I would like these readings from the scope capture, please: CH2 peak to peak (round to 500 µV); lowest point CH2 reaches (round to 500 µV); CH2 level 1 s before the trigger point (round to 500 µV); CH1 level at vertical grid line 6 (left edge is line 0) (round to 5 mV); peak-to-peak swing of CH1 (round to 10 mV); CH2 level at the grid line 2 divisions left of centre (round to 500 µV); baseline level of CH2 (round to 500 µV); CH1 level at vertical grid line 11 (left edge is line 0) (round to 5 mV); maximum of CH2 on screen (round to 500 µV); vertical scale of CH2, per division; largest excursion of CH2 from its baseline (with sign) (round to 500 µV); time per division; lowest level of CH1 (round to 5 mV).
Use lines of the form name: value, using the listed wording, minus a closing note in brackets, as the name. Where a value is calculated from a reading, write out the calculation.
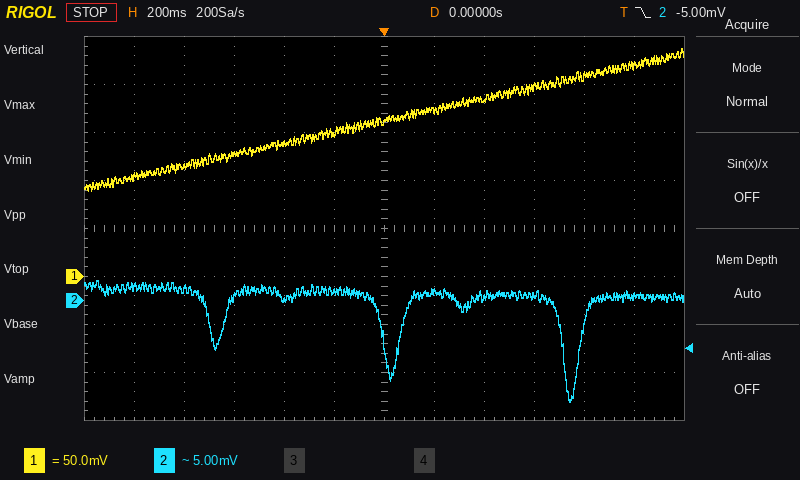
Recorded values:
CH2 peak to peak: 2.0 mV − (-10.5 mV) = 12.5 mV
lowest point CH2 reaches: -10.5 mV
CH2 level 1 s before the trigger point: 1.5 mV
CH1 level at vertical grid line 6 (left edge is line 0): 160 mV
peak-to-peak swing of CH1: 150 mV
CH2 level at the grid line 2 divisions left of centre: 0.0 mV
baseline level of CH2: 500 µV
CH1 level at vertical grid line 11 (left edge is line 0): 220 mV
maximum of CH2 on screen: 2.0 mV
vertical scale of CH2, per division: 5 mV
largest excursion of CH2 from its baseline (with sign): -10.5 mV − (500 µV) = -11.0 mV
time per division: 200 ms
lowest level of CH1: 90 mV
